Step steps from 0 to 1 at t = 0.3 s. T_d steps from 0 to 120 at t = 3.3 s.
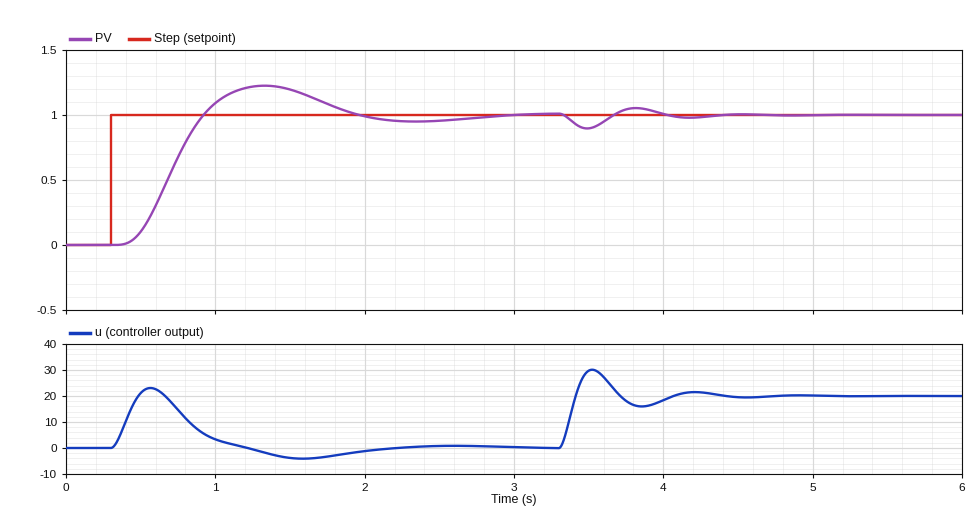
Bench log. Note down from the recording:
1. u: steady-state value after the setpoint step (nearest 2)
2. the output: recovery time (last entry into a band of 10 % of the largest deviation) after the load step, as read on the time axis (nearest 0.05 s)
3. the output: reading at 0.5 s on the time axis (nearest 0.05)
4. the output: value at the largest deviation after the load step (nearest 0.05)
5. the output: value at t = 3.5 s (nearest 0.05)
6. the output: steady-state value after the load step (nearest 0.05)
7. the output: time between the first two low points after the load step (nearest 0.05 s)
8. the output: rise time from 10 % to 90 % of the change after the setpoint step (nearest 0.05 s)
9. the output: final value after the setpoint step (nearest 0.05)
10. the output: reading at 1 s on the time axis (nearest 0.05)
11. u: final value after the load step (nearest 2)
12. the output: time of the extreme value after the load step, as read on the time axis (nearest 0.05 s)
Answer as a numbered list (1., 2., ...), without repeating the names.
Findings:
1. 0
2. 4.30 s
3. 0.10
4. 0.90
5. 0.90
6. 1.00
7. 0.70 s
8. 0.35 s
9. 1.00
10. 1.10
11. 20
12. 3.50 s
